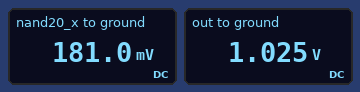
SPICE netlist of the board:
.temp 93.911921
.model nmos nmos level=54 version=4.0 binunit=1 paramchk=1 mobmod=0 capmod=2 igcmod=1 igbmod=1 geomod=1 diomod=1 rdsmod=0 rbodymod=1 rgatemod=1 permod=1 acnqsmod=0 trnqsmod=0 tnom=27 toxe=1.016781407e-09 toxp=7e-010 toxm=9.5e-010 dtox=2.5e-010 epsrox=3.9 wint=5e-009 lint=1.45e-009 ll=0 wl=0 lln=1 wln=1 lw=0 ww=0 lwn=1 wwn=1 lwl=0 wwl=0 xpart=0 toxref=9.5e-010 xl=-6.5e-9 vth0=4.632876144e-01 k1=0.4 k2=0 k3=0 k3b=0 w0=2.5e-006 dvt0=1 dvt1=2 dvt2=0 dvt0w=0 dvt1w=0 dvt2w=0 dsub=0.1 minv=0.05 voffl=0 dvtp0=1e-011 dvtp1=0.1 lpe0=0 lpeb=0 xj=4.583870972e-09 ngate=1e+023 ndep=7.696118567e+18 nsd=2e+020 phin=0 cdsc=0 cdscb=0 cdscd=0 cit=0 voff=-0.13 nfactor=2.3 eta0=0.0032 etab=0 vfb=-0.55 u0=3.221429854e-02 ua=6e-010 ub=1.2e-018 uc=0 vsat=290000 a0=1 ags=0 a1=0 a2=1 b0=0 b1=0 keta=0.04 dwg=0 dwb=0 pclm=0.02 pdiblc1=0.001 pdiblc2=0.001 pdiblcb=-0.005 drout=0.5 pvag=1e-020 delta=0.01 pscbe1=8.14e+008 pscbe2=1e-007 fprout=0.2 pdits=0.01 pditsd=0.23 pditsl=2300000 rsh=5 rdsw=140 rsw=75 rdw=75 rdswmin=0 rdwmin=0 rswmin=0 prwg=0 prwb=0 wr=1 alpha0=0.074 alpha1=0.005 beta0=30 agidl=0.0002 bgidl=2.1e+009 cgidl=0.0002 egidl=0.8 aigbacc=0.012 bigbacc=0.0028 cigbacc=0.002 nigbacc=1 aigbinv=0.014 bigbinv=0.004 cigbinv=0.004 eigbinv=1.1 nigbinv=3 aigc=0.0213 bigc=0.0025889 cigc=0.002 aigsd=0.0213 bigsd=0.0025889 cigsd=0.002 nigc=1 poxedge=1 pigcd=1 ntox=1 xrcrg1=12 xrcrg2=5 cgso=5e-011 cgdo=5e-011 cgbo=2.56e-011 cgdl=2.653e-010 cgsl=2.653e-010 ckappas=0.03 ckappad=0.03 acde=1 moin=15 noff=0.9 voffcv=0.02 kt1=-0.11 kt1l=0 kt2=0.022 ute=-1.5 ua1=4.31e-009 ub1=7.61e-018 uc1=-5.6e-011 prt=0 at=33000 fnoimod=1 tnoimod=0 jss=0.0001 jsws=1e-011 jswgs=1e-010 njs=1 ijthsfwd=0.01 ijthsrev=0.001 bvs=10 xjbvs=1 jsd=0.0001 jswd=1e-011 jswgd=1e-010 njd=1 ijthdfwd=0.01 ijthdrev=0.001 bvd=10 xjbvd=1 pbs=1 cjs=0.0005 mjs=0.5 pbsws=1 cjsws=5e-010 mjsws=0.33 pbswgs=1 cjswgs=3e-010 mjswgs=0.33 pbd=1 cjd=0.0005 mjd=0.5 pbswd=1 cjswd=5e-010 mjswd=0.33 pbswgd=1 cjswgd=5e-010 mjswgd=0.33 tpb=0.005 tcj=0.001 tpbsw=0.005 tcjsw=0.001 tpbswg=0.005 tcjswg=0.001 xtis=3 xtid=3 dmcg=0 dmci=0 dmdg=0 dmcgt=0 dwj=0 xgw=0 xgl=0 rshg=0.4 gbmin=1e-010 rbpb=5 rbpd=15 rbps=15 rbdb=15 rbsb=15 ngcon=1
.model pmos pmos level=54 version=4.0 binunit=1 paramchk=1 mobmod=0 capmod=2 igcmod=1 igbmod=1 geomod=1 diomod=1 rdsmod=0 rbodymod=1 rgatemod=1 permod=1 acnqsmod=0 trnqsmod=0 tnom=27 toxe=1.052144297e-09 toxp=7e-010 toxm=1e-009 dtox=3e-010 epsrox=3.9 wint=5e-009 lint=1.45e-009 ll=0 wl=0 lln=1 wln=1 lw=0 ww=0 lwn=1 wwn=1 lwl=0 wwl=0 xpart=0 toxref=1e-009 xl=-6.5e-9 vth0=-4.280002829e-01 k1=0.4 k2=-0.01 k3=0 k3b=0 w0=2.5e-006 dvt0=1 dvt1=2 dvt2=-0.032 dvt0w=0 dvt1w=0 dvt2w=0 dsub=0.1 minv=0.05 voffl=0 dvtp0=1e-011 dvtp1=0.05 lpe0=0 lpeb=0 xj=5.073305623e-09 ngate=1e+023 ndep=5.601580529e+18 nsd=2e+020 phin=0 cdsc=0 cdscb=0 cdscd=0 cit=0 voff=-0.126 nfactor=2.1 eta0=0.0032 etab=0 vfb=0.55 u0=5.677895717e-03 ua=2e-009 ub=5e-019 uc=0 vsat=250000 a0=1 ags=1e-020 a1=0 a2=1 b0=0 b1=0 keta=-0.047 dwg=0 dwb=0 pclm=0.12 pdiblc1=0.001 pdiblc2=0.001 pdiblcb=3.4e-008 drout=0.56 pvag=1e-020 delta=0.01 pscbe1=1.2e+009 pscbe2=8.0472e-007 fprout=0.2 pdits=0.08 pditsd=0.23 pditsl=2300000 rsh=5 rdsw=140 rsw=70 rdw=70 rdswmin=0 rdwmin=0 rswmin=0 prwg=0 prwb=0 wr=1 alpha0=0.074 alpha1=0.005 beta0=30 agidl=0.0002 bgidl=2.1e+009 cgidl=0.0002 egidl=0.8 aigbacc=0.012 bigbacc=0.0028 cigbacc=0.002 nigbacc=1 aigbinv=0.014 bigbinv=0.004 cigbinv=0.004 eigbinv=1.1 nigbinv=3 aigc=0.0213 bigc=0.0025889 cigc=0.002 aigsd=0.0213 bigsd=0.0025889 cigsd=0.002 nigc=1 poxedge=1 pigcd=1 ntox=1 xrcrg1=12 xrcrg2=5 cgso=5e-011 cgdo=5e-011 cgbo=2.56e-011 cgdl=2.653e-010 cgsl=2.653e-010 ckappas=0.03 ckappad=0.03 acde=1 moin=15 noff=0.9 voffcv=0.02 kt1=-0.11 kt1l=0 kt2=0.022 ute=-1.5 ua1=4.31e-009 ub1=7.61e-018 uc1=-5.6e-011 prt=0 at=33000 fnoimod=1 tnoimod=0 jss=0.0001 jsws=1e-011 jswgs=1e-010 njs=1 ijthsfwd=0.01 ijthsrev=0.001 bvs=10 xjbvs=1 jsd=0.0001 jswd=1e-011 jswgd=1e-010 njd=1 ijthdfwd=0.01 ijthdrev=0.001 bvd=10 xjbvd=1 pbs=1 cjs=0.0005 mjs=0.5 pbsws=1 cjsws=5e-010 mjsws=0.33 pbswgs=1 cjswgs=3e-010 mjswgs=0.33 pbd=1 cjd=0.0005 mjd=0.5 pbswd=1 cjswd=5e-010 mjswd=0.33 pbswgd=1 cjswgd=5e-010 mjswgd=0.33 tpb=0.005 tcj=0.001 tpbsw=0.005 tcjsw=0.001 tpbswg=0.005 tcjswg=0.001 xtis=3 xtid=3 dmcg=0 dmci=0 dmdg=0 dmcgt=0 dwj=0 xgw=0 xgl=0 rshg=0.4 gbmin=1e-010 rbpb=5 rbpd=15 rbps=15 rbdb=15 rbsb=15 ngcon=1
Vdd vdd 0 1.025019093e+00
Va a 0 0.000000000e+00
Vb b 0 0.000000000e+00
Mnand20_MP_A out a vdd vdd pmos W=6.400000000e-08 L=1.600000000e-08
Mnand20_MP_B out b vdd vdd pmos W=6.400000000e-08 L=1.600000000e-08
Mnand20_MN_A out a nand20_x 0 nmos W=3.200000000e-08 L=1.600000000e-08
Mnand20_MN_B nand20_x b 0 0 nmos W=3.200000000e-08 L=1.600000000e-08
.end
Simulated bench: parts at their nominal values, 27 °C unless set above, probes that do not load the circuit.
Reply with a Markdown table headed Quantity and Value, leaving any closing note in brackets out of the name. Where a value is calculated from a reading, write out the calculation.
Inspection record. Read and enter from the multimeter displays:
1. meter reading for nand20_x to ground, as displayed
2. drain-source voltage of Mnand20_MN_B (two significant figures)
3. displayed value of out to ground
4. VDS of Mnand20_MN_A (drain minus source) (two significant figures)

| Quantity | Value |
|---|---|
| meter reading for nand20_x to ground, as displayed | 181.0 mV |
| drain-source voltage of Mnand20_MN_B | 181 mV = 180 mV |
| displayed value of out to ground | 1.025 V |
| VDS of Mnand20_MN_A (drain minus source) | 1.025 V - 181 mV = 840 mV |
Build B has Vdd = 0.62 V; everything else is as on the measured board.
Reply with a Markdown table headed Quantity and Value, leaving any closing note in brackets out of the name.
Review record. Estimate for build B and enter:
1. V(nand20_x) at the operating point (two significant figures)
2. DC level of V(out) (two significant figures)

| Quantity | Value |
|---|---|
| V(nand20_x) at the operating point | 110 mV |
| DC level of V(out) | 620 mV |
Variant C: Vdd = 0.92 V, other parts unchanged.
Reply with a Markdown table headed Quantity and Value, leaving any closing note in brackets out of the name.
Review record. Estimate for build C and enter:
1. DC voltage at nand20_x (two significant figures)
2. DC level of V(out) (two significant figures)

| Quantity | Value |
|---|---|
| DC voltage at nand20_x | 160 mV |
| DC level of V(out) | 920 mV |
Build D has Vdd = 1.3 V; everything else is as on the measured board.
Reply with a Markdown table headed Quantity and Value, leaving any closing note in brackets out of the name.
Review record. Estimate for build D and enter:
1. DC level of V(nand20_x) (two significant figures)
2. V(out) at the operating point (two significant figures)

| Quantity | Value |
|---|---|
| DC level of V(nand20_x) | 240 mV |
| V(out) at the operating point | 1.3 V |
